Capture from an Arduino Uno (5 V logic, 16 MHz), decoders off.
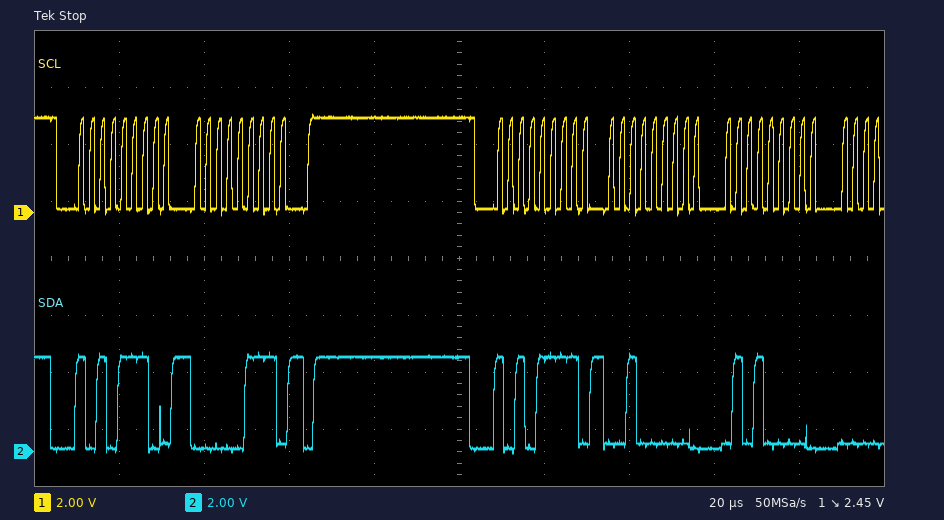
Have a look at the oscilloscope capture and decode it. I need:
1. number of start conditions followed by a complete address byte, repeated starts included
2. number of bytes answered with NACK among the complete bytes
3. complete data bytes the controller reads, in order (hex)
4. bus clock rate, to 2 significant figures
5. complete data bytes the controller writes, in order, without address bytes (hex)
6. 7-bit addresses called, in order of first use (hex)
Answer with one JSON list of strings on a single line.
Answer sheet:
["2", "0", "20 50", "400 kHz", "07", "0x57"]
